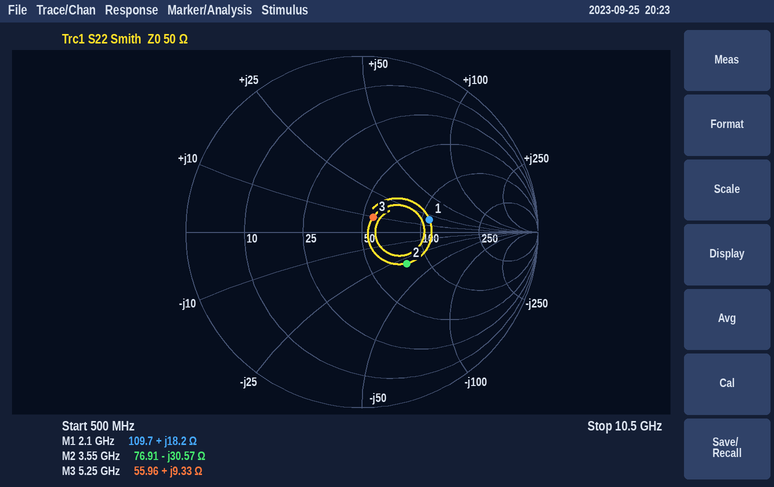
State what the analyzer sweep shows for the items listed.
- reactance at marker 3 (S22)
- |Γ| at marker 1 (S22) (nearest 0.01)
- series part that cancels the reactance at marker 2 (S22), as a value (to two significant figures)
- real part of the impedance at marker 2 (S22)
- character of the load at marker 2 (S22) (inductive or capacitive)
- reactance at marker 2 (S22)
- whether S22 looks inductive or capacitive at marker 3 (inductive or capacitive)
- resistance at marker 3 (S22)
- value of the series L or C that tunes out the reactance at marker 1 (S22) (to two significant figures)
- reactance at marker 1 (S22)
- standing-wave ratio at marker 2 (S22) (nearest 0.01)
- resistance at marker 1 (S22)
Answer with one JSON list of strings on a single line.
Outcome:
["+9.33 Ω", "0.39", "1.4 nH", "76.91 Ω", "capacitive", "-30.57 Ω", "inductive", "55.96 Ω", "4.2 pF", "+18.2 Ω", "1.91", "109.7 Ω"]
